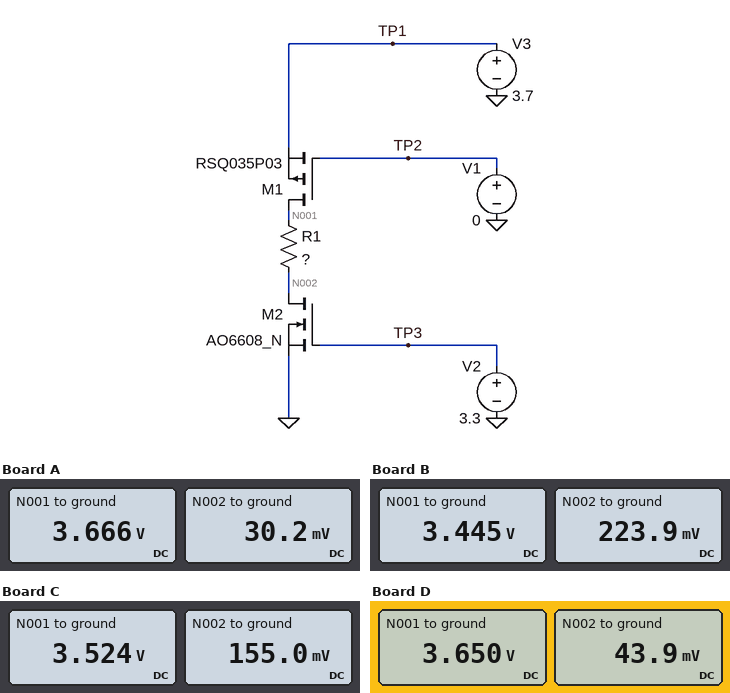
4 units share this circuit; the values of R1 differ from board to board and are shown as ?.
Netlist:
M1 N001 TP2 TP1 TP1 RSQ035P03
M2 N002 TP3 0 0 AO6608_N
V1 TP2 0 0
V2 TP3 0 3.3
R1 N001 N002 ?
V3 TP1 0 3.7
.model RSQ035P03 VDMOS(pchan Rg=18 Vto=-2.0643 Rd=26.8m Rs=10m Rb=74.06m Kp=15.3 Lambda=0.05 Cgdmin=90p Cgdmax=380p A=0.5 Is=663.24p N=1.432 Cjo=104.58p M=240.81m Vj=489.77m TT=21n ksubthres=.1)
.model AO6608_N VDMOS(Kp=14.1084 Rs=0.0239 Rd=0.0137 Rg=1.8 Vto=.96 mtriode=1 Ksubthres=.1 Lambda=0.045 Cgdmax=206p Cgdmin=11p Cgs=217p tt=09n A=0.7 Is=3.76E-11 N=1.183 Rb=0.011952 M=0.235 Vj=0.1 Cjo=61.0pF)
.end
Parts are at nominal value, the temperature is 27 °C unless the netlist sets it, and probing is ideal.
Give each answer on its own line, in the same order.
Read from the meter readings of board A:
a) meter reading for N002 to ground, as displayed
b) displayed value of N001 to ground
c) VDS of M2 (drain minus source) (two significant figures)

30.2 mV
3.666 V
30 mV
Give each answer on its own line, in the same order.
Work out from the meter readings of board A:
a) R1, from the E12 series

8.2 Ω
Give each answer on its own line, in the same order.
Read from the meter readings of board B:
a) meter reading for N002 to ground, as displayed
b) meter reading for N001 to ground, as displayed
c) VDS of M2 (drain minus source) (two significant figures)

223.9 mV
3.445 V
220 mV
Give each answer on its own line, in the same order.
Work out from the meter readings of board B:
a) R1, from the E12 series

1 Ω
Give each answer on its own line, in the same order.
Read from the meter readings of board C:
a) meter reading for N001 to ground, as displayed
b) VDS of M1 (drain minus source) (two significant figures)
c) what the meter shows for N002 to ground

3.524 V
-180 mV
155.0 mV
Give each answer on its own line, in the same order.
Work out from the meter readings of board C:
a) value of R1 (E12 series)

1.5 Ω
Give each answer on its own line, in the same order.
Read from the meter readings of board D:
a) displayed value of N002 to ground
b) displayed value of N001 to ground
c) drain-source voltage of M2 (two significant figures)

43.9 mV
3.650 V
44 mV
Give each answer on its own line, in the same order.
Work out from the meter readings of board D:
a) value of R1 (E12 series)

5.6 Ω
